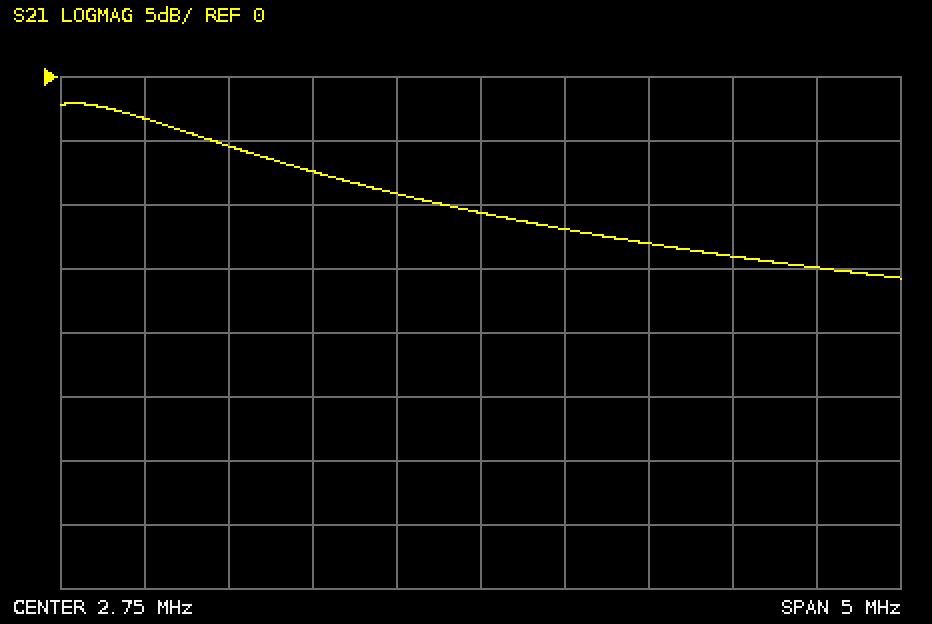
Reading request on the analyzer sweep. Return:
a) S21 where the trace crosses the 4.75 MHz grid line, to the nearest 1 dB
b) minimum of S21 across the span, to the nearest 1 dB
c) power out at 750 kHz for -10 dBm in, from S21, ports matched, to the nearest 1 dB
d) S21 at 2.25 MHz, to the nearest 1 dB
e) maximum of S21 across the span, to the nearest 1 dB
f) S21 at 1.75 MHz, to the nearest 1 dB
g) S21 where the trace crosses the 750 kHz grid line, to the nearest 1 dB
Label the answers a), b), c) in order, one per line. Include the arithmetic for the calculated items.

a) -15 dB
b) -16 dB
c) -10 dBm + (-3 dB) = -13 dBm
d) -9 dB
e) -2 dB
f) -7 dB
g) -3 dB
